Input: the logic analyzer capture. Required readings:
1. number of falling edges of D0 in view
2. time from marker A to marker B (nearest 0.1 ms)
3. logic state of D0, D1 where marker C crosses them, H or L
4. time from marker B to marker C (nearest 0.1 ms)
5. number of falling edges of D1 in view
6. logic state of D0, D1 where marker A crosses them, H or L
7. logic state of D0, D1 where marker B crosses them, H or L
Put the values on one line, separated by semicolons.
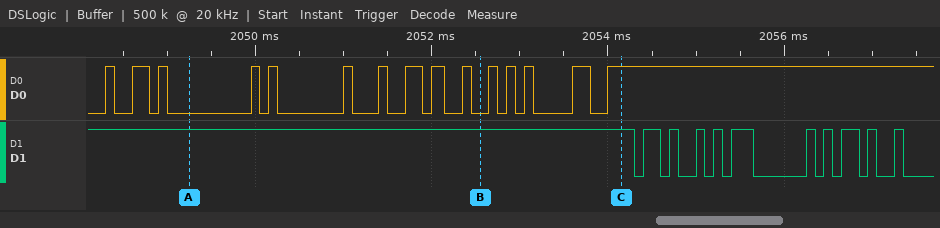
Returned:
14; 3.3 ms; D0=H, D1=H; 1.6 ms; 11; D0=L, D1=H; D0=L, D1=H
